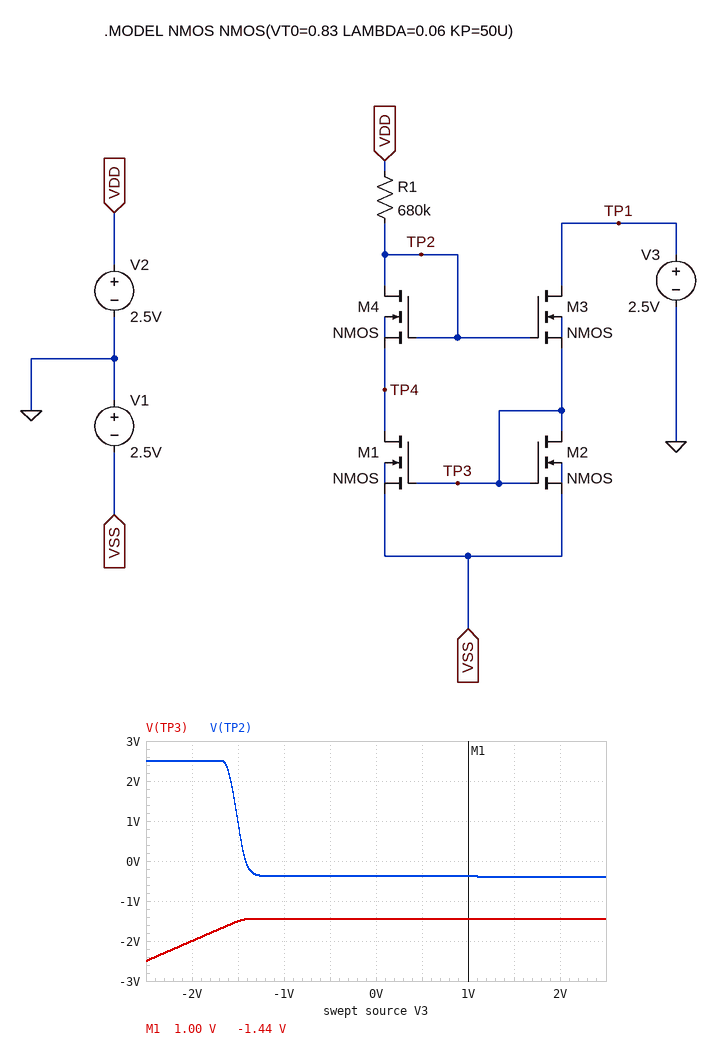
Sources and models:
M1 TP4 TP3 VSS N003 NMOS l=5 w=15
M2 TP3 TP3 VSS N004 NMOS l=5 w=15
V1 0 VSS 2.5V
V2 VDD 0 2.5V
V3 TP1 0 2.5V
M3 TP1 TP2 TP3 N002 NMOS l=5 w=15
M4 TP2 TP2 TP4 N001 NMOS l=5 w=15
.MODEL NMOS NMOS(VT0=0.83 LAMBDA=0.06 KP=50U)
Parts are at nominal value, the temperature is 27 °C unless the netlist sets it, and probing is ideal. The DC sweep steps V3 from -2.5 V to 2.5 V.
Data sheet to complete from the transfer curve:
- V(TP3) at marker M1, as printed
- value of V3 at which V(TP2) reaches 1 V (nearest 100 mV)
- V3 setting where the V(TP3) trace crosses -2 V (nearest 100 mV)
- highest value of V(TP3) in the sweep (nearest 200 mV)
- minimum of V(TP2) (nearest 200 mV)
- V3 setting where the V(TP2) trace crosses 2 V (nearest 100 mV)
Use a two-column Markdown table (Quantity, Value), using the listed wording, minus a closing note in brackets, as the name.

| Quantity | Value |
|---|---|
| V(TP3) at marker M1, as printed | -1.44 V |
| value of V3 at which V(TP2) reaches 1 V | -1.5 V |
| V3 setting where the V(TP3) trace crosses -2 V | -2.0 V |
| highest value of V(TP3) in the sweep | -1.4 V |
| minimum of V(TP2) | -400 mV |
| V3 setting where the V(TP2) trace crosses 2 V | -1.6 V |
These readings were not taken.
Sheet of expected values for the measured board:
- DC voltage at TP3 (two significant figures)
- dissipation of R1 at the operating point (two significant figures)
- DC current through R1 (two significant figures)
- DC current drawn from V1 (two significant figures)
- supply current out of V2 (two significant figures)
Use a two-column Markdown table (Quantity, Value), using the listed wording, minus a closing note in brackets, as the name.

| Quantity | Value |
|---|---|
| DC voltage at TP3 | -1.4 V |
| dissipation of R1 at the operating point | 12 µW |
| DC current through R1 | 4.3 µA |
| DC current drawn from V1 | 8.5 µA |
| supply current out of V2 | 4.3 µA |
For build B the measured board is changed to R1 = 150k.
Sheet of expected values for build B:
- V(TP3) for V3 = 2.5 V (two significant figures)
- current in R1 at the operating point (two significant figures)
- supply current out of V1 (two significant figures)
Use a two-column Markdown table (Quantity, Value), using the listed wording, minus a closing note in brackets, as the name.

| Quantity | Value |
|---|---|
| V(TP3) for V3 = 2.5 V | -1.2 V |
| current in R1 at the operating point | 16 µA |
| supply current out of V1 | 33 µA |
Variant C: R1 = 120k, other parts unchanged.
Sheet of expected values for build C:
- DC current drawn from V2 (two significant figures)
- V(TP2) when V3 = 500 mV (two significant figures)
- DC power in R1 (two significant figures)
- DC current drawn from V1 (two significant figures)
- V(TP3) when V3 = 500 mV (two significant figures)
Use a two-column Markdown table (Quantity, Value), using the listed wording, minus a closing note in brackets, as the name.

| Quantity | Value |
|---|---|
| DC current drawn from V2 | 20 µA |
| V(TP2) when V3 = 500 mV | 140 mV |
| DC power in R1 | 47 µW |
| DC current drawn from V1 | 40 µA |
| V(TP3) when V3 = 500 mV | -1.2 V |
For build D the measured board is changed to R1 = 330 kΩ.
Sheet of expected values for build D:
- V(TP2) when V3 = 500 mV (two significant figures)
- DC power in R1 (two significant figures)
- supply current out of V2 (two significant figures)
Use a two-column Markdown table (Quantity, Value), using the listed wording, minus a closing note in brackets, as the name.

| Quantity | Value |
|---|---|
| V(TP2) when V3 = 500 mV | -210 mV |
| DC power in R1 | 22 µW |
| supply current out of V2 | 8.2 µA |
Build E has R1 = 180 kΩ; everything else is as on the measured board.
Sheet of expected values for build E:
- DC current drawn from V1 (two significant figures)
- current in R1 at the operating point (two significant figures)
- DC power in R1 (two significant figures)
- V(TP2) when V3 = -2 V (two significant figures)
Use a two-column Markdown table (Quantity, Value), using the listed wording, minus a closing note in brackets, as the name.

| Quantity | Value |
|---|---|
| DC current drawn from V1 | 28 µA |
| current in R1 at the operating point | 14 µA |
| DC power in R1 | 36 µW |
| V(TP2) when V3 = -2 V | 2.5 V |
